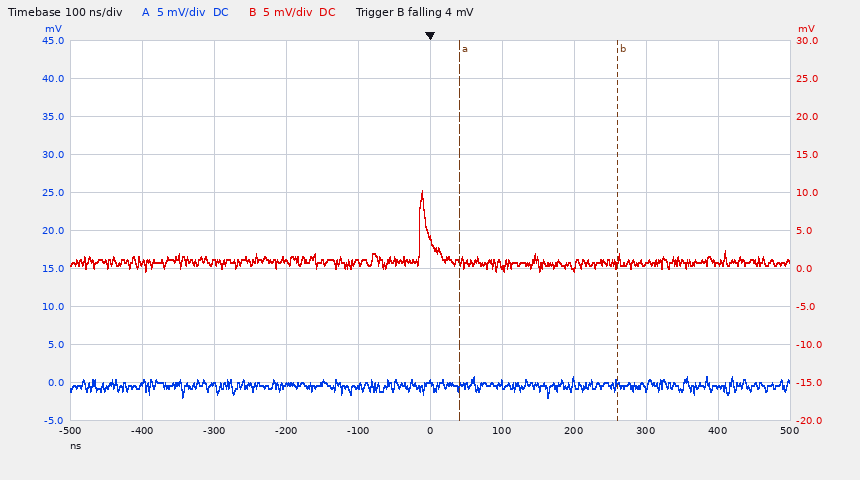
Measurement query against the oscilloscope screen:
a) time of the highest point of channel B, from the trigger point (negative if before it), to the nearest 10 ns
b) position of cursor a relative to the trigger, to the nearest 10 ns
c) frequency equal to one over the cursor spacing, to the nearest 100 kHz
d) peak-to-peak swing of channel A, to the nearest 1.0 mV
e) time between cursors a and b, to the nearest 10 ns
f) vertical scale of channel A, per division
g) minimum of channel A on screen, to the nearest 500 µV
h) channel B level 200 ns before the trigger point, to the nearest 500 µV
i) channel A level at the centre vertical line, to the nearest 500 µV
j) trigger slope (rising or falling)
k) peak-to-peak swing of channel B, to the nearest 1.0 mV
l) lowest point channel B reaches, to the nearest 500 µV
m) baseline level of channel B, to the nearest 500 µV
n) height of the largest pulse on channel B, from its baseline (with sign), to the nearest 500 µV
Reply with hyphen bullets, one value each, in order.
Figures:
- -10 ns
- +40 ns
- 4.5 MHz
- 3.0 mV
- 220 ns
- 5 mV
- -2.0 mV
- 1.0 mV
- 0.0 mV
- falling
- 11.0 mV
- -500 µV
- 1.0 mV
- +9.5 mV
